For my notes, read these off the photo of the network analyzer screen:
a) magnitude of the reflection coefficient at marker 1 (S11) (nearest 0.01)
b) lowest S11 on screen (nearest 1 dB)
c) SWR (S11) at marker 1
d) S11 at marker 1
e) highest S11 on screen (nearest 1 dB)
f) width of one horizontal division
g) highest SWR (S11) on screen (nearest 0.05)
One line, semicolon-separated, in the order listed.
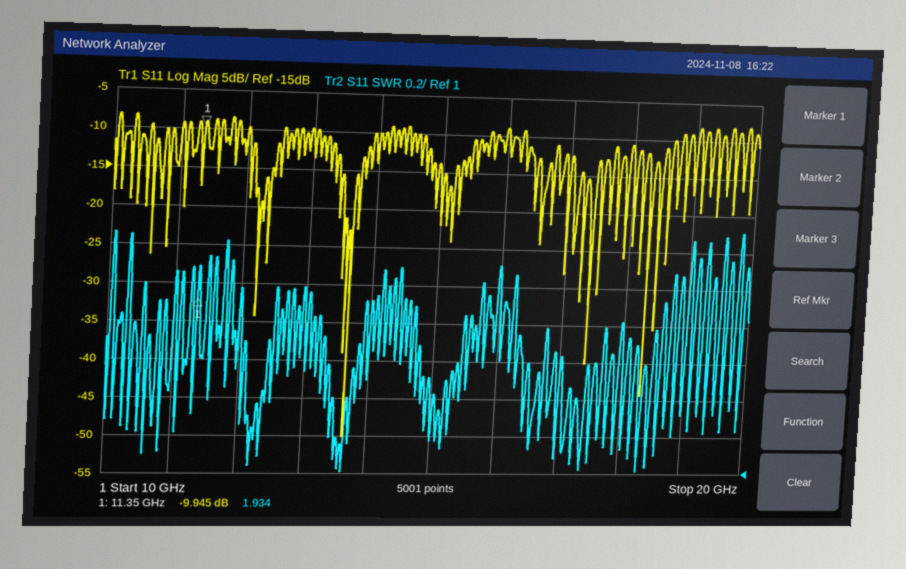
0.32; -50 dB; 1.934; -9.945 dB; -8 dB; 1 GHz; 2.30
